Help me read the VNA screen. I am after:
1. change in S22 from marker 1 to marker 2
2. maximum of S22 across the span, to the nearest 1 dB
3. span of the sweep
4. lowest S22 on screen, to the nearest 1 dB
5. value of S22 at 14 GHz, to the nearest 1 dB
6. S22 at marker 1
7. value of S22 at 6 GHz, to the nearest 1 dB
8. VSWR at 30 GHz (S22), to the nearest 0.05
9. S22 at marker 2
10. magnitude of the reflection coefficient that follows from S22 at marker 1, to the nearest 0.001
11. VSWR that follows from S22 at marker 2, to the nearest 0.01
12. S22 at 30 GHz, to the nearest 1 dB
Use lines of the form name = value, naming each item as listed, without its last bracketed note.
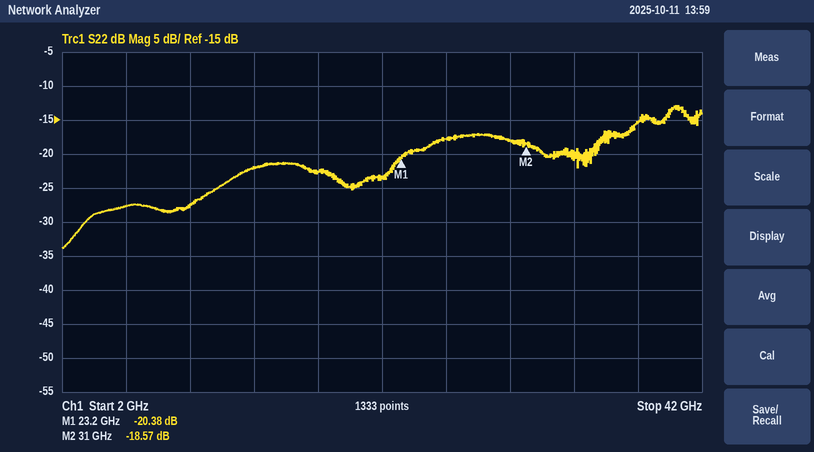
change in S22 from marker 1 to marker 2 = 1.81 dB
maximum of S22 across the span, to the nearest 1 dB = -13 dB
span of the sweep = 40 GHz
lowest S22 on screen, to the nearest 1 dB = -34 dB
value of S22 at 14 GHz, to the nearest 1 dB = -22 dB
S22 at marker 1 = -20.38 dB
value of S22 at 6 GHz, to the nearest 1 dB = -28 dB
VSWR at 30 GHz (S22), to the nearest 0.05 = 1.30
S22 at marker 2 = -18.57 dB
magnitude of the reflection coefficient that follows from S22 at marker 1, to the nearest 0.001 = 0.096
VSWR that follows from S22 at marker 2, to the nearest 0.01 = 1.27
S22 at 30 GHz, to the nearest 1 dB = -18 dB
